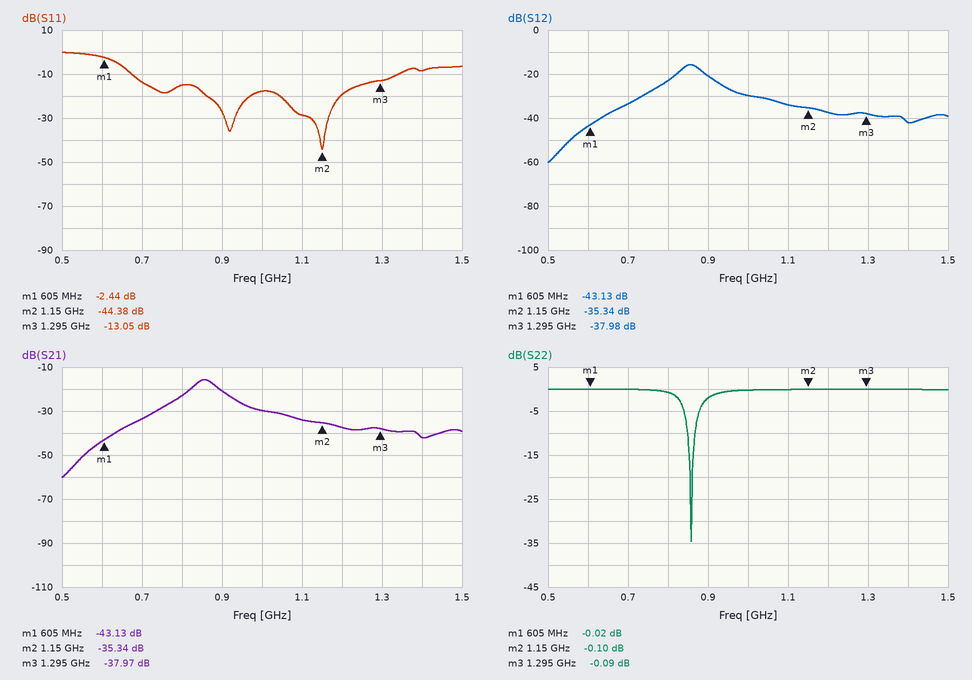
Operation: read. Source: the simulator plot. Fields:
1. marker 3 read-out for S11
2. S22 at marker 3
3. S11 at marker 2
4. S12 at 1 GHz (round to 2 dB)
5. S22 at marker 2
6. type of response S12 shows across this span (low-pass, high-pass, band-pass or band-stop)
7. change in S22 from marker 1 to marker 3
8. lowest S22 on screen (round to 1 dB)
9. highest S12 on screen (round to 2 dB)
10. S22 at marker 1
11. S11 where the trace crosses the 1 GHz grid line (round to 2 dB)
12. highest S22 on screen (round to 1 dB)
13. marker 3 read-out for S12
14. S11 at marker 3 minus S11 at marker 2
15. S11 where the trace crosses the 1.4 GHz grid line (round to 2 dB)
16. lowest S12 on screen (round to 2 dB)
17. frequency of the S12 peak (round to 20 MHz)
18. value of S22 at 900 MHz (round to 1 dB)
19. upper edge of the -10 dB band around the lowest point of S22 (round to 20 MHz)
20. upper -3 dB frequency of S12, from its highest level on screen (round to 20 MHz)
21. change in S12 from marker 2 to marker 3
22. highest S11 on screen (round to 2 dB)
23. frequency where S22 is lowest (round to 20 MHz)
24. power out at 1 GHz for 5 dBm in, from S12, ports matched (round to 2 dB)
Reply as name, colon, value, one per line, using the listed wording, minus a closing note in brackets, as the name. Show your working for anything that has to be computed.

marker 3 read-out for S11: -13.05 dB
S22 at marker 3: -0.09 dB
S11 at marker 2: -44.38 dB
S12 at 1 GHz: -30 dB
S22 at marker 2: -0.10 dB
type of response S12 shows across this span: band-pass
change in S22 from marker 1 to marker 3: -0.09 − (-0.02) = -0.07 dB
lowest S22 on screen: -35 dB
highest S12 on screen: -16 dB
S22 at marker 1: -0.02 dB
S11 where the trace crosses the 1 GHz grid line: -18 dB
highest S22 on screen: 0 dB
marker 3 read-out for S12: -37.98 dB
S11 at marker 3 minus S11 at marker 2: -13.05 − (-44.38) = 31.33 dB
S11 where the trace crosses the 1.4 GHz grid line: -8 dB
lowest S12 on screen: -60 dB
frequency of the S12 peak: 860 MHz
value of S22 at 900 MHz: -2 dB
upper edge of the -10 dB band around the lowest point of S22: 860 MHz
upper -3 dB frequency of S12, from its highest level on screen: 880 MHz
change in S12 from marker 2 to marker 3: -37.98 − (-35.34) = -2.64 dB
highest S11 on screen: 0 dB
frequency where S22 is lowest: 860 MHz
power out at 1 GHz for 5 dBm in, from S12, ports matched: 5 dBm + (-30 dB) = -24 dBm
